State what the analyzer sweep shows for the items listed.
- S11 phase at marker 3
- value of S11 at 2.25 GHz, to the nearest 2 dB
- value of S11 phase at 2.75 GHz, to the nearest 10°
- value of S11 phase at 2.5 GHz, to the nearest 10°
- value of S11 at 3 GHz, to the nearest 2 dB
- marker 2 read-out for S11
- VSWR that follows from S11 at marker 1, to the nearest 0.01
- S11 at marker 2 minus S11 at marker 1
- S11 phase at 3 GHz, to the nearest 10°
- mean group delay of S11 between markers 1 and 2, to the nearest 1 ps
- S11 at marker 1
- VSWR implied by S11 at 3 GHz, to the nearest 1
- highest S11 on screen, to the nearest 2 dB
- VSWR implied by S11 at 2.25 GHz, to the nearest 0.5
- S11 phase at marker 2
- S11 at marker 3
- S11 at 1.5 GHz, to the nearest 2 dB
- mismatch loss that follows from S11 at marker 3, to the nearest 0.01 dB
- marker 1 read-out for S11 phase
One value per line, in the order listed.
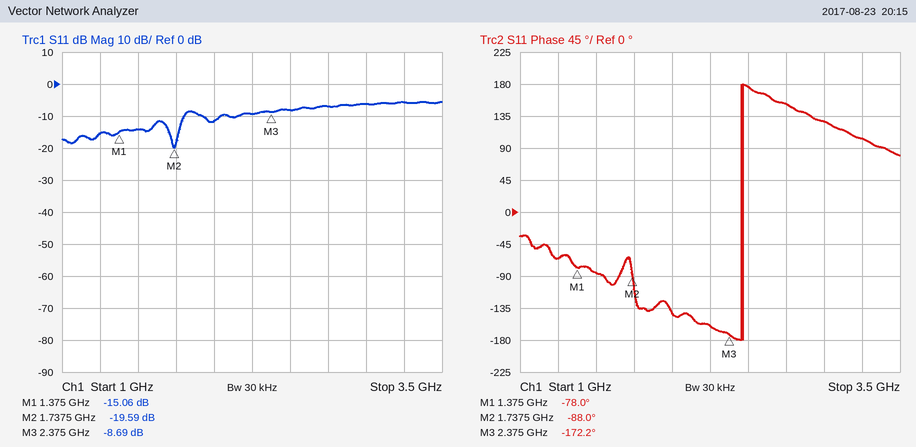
-172.2°
-10 dB
150°
180°
-6 dB
-19.59 dB
1.43
-4.53 dB
130°
77 ps
-15.06 dB
3
-6 dB
2.0
-88.0°
-8.69 dB
-14 dB
0.63 dB
-78.0°
